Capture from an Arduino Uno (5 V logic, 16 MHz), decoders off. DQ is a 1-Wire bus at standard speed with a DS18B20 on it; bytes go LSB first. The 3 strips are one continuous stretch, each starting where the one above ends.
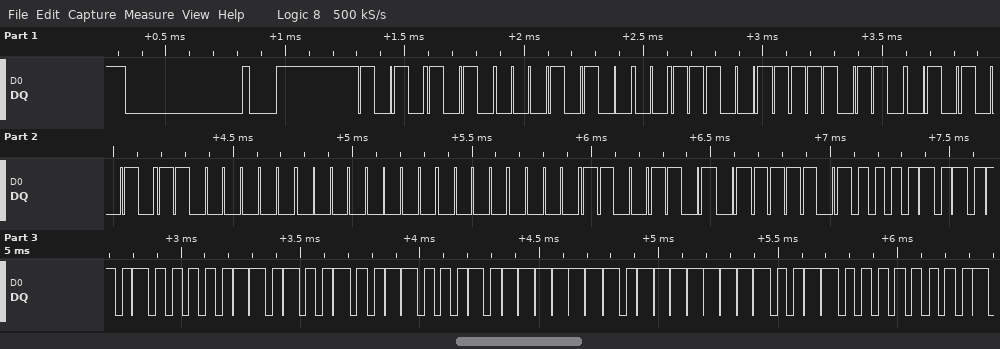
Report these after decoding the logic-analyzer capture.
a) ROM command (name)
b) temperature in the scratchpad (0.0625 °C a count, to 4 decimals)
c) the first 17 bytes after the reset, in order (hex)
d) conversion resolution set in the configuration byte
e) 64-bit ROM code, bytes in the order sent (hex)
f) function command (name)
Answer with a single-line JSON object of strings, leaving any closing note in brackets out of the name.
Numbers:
{"ROM command": "Match ROM", "temperature in the scratchpad": "85.0000 °C", "the first 17 bytes after the reset, in order": "55 28 9C 6F 4A 03 00 00 B3 BE 50 05 4B 46 7F FF 0C", "conversion resolution set in the configuration byte": "12 bits", "64-bit ROM code, bytes in the order sent": "28 9C 6F 4A 03 00 00 B3", "function command": "Read Scratchpad"}
